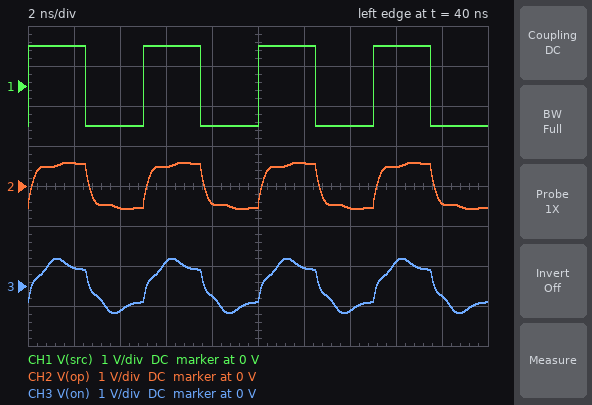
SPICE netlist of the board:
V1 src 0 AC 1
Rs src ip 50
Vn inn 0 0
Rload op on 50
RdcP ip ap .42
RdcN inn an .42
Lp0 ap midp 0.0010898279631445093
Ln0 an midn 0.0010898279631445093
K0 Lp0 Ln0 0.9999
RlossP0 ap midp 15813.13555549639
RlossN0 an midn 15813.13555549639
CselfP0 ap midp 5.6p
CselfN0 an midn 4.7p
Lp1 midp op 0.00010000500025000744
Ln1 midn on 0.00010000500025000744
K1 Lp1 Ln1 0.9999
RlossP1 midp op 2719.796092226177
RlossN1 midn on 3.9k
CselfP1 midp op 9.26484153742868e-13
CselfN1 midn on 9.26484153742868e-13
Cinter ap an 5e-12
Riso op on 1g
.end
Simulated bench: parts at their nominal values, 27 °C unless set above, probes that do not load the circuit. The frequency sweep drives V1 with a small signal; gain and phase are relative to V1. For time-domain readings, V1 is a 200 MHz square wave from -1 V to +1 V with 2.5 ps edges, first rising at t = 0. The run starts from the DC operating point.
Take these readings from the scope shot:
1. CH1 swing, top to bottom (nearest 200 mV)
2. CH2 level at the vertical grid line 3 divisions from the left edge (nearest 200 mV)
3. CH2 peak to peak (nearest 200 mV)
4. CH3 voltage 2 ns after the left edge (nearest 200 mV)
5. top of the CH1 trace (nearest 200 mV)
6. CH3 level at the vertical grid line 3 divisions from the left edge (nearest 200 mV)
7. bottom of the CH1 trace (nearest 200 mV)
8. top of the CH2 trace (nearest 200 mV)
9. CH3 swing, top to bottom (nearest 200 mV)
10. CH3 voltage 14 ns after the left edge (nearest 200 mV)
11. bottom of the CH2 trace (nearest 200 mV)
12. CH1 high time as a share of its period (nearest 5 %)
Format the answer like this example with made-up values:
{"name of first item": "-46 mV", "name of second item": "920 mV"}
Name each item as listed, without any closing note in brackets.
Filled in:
{"CH1 swing, top to bottom": "2.0 V", "CH2 level at the vertical grid line 3 divisions from the left edge": "400 mV", "CH2 peak to peak": "1.2 V", "CH3 voltage 2 ns after the left edge": "400 mV", "top of the CH1 trace": "1.0 V", "CH3 level at the vertical grid line 3 divisions from the left edge": "600 mV", "bottom of the CH1 trace": "-1.0 V", "top of the CH2 trace": "600 mV", "CH3 swing, top to bottom": "1.4 V", "CH3 voltage 14 ns after the left edge": "-600 mV", "bottom of the CH2 trace": "-600 mV", "CH1 high time as a share of its period": "50 %"}
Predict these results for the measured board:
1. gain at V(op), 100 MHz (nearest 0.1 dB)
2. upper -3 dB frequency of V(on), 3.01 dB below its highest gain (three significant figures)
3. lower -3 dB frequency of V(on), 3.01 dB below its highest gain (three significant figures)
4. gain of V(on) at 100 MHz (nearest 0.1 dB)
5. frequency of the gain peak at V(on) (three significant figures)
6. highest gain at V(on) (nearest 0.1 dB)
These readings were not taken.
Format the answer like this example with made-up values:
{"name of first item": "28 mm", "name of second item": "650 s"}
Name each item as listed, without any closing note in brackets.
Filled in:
{"gain at V(op), 100 MHz": "-5.3 dB", "upper -3 dB frequency of V(on), 3.01 dB below its highest gain": "399 MHz", "lower -3 dB frequency of V(on), 3.01 dB below its highest gain": "57.1 MHz", "gain of V(on) at 100 MHz": "-6.2 dB", "frequency of the gain peak at V(on)": "162 MHz", "highest gain at V(on)": "-5.6 dB"}
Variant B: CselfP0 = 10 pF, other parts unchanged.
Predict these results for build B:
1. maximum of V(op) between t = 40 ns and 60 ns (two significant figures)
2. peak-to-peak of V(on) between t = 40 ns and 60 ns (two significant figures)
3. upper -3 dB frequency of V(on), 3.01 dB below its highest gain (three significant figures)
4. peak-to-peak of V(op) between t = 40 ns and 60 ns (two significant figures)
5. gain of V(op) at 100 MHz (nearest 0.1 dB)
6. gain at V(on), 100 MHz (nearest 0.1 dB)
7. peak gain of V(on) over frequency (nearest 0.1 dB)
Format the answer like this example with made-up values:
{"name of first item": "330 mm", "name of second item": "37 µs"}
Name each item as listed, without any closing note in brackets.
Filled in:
{"maximum of V(op) between t = 40 ns and 60 ns": "690 mV", "peak-to-peak of V(on) between t = 40 ns and 60 ns": "1.7 V", "upper -3 dB frequency of V(on), 3.01 dB below its highest gain": "380 MHz", "peak-to-peak of V(op) between t = 40 ns and 60 ns": "1.4 V", "gain of V(op) at 100 MHz": "-3.7 dB", "gain at V(on), 100 MHz": "-4.3 dB", "peak gain of V(on) over frequency": "-3.6 dB"}
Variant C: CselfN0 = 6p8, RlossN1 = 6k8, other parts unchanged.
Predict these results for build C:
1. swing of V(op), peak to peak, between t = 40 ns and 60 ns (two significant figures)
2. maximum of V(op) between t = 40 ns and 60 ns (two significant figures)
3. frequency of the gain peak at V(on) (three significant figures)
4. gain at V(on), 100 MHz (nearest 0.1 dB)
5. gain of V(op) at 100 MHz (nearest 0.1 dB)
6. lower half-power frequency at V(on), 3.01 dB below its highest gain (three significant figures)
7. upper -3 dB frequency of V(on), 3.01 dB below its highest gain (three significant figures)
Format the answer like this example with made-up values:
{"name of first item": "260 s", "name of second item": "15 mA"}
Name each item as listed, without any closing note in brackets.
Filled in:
{"swing of V(op), peak to peak, between t = 40 ns and 60 ns": "1.0 V", "maximum of V(op) between t = 40 ns and 60 ns": "510 mV", "frequency of the gain peak at V(on)": "150 MHz", "gain at V(on), 100 MHz": "-7.6 dB", "gain of V(op) at 100 MHz": "-6.4 dB", "lower half-power frequency at V(on), 3.01 dB below its highest gain": "55.3 MHz", "upper -3 dB frequency of V(on), 3.01 dB below its highest gain": "342 MHz"}
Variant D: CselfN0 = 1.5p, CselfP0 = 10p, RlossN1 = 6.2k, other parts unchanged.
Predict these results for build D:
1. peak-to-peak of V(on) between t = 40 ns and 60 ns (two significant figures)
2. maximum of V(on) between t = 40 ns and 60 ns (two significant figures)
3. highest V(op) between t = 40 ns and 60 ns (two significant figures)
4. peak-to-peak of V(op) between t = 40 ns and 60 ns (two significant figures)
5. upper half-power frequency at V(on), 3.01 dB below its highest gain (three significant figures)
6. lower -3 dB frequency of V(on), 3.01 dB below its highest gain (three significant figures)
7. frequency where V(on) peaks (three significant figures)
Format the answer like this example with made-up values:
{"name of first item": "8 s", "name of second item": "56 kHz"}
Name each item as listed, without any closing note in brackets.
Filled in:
{"peak-to-peak of V(on) between t = 40 ns and 60 ns": "2.2 V", "maximum of V(on) between t = 40 ns and 60 ns": "1.1 V", "highest V(op) between t = 40 ns and 60 ns": "950 mV", "peak-to-peak of V(op) between t = 40 ns and 60 ns": "1.9 V", "upper half-power frequency at V(on), 3.01 dB below its highest gain": "696 MHz", "lower -3 dB frequency of V(on), 3.01 dB below its highest gain": "58.7 MHz", "frequency where V(on) peaks": "191 MHz"}
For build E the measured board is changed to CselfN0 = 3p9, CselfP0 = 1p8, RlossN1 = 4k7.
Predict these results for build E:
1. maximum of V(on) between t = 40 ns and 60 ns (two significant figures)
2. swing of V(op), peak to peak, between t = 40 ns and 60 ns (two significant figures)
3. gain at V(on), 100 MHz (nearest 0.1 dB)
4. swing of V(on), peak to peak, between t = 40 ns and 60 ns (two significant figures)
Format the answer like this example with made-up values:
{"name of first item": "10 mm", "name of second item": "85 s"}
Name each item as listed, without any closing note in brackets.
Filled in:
{"maximum of V(on) between t = 40 ns and 60 ns": "460 mV", "swing of V(op), peak to peak, between t = 40 ns and 60 ns": "900 mV", "gain at V(on), 100 MHz": "-10.7 dB", "swing of V(on), peak to peak, between t = 40 ns and 60 ns": "920 mV"}
